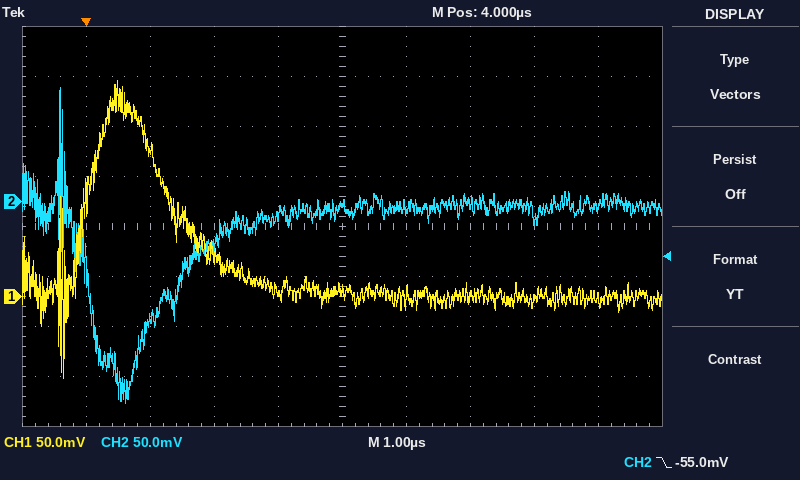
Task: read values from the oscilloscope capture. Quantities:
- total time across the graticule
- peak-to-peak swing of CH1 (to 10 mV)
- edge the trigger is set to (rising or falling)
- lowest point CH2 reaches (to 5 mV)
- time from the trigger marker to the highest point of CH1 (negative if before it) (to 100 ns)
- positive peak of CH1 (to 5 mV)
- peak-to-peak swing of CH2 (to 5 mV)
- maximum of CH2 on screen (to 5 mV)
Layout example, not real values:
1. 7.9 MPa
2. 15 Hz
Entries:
1. 10 µs
2. 300 mV
3. falling
4. -200 mV
5. +500 ns
6. 215 mV
7. 315 mV
8. 115 mV
